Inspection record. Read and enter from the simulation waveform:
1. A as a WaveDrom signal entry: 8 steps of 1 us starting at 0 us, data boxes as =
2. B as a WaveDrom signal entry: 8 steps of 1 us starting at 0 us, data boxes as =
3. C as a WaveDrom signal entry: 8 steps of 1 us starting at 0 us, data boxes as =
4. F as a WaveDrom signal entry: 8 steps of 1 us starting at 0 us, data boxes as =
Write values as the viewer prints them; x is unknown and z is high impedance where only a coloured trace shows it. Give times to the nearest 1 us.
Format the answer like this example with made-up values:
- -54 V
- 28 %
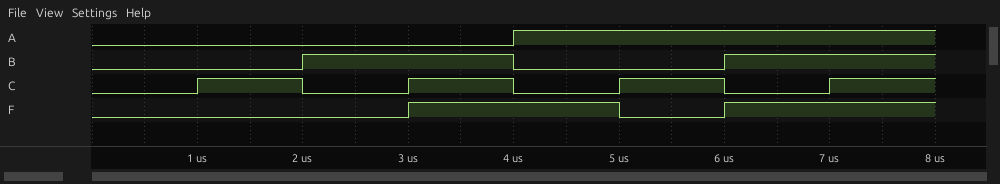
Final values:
- {name: 'A', wave: '0...1...'}
- {name: 'B', wave: '0.1.0.1.'}
- {name: 'C', wave: '01010101'}
- {name: 'F', wave: '0..1.01.'}
